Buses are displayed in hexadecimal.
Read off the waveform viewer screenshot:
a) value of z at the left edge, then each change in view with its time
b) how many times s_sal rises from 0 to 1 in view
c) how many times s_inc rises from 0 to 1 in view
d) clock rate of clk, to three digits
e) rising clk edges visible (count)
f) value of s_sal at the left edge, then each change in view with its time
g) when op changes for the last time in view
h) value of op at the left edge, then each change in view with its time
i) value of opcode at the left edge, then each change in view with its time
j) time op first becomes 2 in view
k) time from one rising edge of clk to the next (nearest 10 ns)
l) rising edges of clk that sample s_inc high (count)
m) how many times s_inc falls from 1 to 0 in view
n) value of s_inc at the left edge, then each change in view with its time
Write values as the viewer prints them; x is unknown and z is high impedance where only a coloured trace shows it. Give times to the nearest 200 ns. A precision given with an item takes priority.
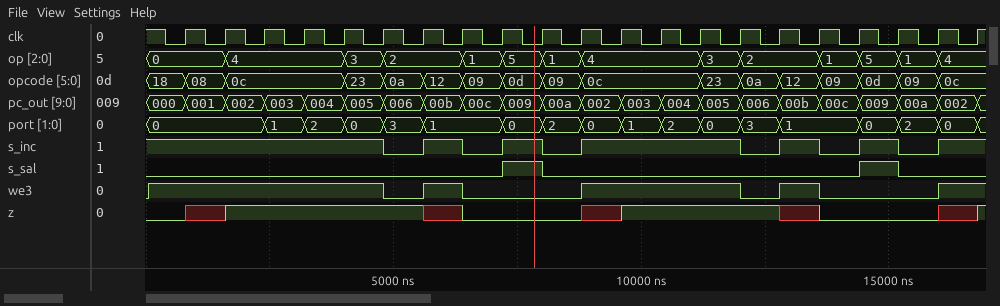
0, x at 800 ns, 1 at 1600 ns, x at 5600 ns, 0 at 6400 ns, x at 8800 ns, 1 at 9600 ns, x at 12800 ns, 0 at 13600 ns, x at 16000 ns, 1 at 16800 ns
2
6
1.25 MHz
21
0, 1 at 7200 ns, 0 at 8000 ns, 1 at 14400 ns, 0 at 15200 ns
16000 ns
0, 4 at 1600 ns, 3 at 4000 ns, 2 at 4800 ns, 1 at 6400 ns, 5 at 7200 ns, 1 at 8000 ns, 4 at 8800 ns, 3 at 11200 ns, 2 at 12000 ns, 1 at 13600 ns, 5 at 14400 ns, 1 at 15200 ns, 4 at 16000 ns
18, 08 at 800 ns, 0c at 1600 ns, 23 at 4000 ns, 0a at 4800 ns, 12 at 5600 ns, 09 at 6400 ns, 0d at 7200 ns, 09 at 8000 ns, 0c at 8800 ns, 23 at 11200 ns, 0a at 12000 ns, 12 at 12800 ns, 09 at 13600 ns, 0d at 14400 ns, 09 at 15200 ns, 0c at 16000 ns
4800 ns
800 ns
15
6
1, 0 at 4800 ns, 1 at 5600 ns, 0 at 6400 ns, 1 at 7200 ns, 0 at 8000 ns, 1 at 8800 ns, 0 at 12000 ns, 1 at 12800 ns, 0 at 13600 ns, 1 at 14400 ns, 0 at 15200 ns, 1 at 16000 ns
